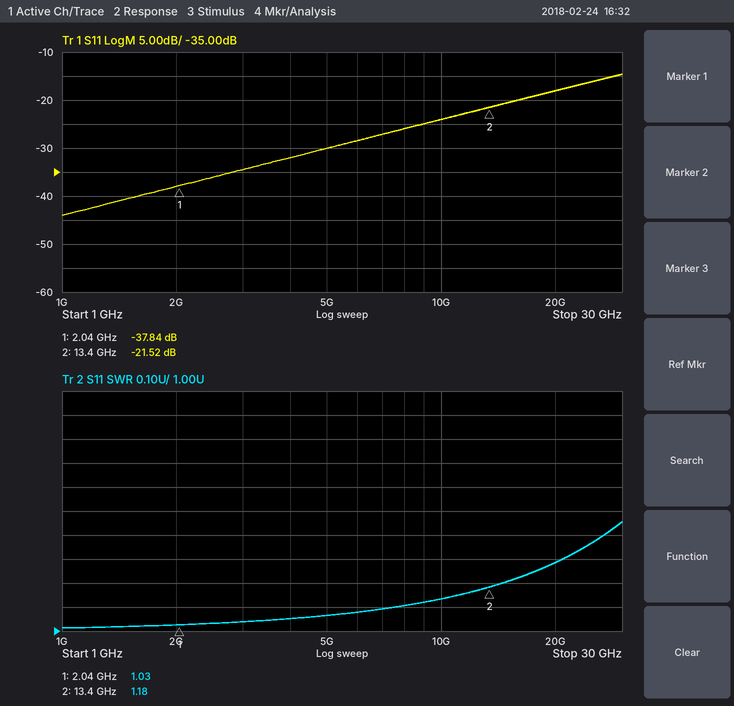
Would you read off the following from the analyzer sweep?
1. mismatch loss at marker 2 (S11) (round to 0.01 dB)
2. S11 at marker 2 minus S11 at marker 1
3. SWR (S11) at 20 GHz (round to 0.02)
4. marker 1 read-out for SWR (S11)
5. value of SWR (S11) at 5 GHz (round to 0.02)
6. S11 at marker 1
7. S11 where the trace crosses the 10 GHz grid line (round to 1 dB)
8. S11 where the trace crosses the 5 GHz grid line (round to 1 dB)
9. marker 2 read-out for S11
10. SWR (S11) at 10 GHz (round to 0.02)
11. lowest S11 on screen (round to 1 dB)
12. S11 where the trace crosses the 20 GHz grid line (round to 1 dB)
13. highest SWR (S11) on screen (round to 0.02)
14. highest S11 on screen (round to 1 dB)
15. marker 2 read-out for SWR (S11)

0.03 dB
16.32 dB
1.28
1.03
1.06
-37.84 dB
-24 dB
-30 dB
-21.52 dB
1.14
-44 dB
-18 dB
1.46
-15 dB
1.18
